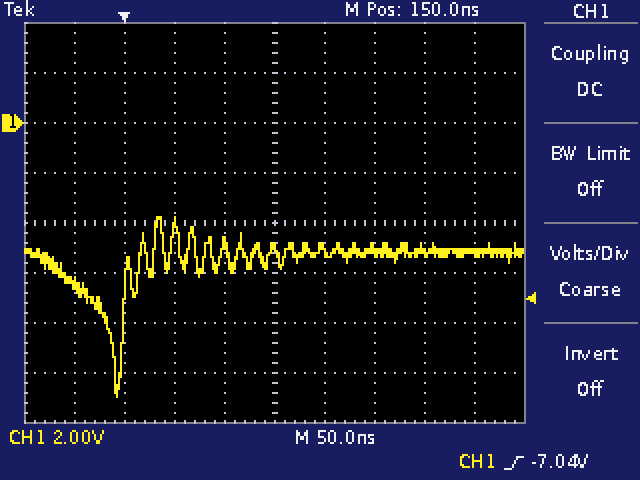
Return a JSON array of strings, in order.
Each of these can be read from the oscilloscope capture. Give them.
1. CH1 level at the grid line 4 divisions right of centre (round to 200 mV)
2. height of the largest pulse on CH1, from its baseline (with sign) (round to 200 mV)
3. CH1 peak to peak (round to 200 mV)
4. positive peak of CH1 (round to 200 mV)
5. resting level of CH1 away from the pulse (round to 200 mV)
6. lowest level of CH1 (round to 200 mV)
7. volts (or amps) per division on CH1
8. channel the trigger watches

["-5.2 V", "-5.8 V", "7.2 V", "-3.8 V", "-5.2 V", "-11.0 V", "2 V", "CH1"]
